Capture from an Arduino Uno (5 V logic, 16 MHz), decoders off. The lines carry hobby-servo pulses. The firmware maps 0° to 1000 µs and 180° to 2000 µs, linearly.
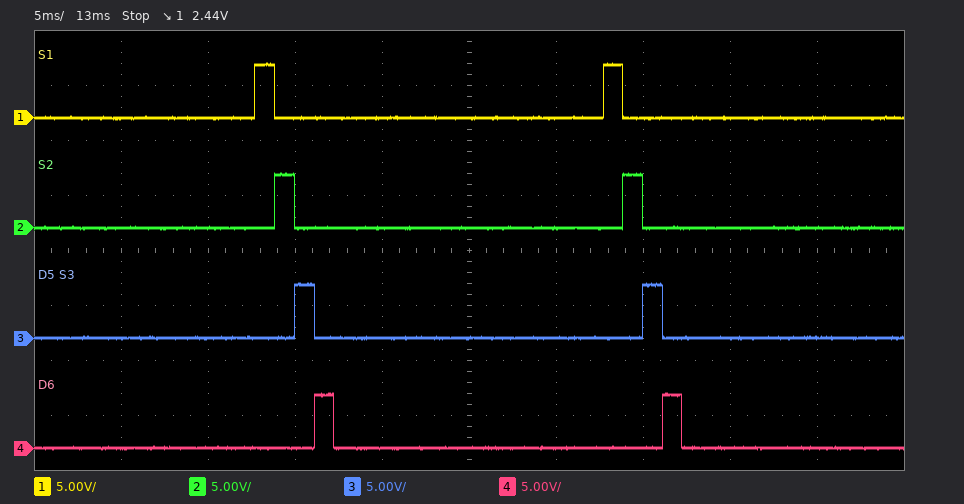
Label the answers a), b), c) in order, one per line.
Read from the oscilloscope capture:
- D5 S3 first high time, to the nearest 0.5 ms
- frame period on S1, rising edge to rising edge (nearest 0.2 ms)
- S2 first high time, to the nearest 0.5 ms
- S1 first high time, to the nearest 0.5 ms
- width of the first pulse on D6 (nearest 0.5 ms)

a) 1.0 ms
b) 20.0 ms
c) 1.0 ms
d) 1.0 ms
e) 1.0 ms
